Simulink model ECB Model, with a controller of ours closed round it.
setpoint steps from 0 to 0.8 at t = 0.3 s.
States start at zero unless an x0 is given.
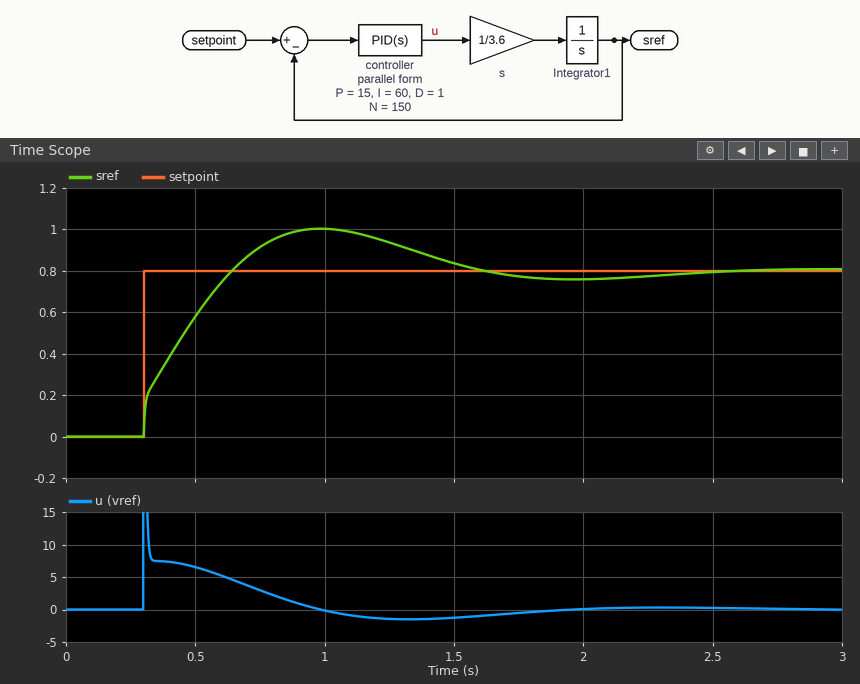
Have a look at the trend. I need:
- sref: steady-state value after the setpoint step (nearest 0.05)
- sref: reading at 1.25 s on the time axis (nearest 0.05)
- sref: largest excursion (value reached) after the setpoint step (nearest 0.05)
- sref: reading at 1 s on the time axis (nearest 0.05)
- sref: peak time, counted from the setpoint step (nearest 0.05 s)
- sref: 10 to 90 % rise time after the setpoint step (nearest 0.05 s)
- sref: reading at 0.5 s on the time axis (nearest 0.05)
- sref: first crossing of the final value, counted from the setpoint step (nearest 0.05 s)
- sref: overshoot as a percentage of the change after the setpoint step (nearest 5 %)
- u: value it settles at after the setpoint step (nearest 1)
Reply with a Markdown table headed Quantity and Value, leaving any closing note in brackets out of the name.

| Quantity | Value |
|---|---|
| sref: steady-state value after the setpoint step | 0.80 |
| sref: reading at 1.25 s on the time axis | 0.95 |
| sref: largest excursion (value reached) after the setpoint step | 1.00 |
| sref: reading at 1 s on the time axis | 1.00 |
| sref: peak time, counted from the setpoint step | 0.70 s |
| sref: 10 to 90 % rise time after the setpoint step | 0.30 s |
| sref: reading at 0.5 s on the time axis | 0.60 |
| sref: first crossing of the final value, counted from the setpoint step | 0.35 s |
| sref: overshoot as a percentage of the change after the setpoint step | 25 % |
| u: value it settles at after the setpoint step | 0 |
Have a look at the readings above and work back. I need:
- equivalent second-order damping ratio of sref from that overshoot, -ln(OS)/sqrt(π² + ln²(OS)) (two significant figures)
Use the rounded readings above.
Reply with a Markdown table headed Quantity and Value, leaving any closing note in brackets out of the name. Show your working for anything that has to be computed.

| Quantity | Value |
|---|---|
| equivalent second-order damping ratio of sref from that overshoot, -ln(OS)/sqrt(π² + ln²(OS)) | ln(0.25) = -1.386; 1.386 / sqrt(9.870 + 1.922) = 0.40 |
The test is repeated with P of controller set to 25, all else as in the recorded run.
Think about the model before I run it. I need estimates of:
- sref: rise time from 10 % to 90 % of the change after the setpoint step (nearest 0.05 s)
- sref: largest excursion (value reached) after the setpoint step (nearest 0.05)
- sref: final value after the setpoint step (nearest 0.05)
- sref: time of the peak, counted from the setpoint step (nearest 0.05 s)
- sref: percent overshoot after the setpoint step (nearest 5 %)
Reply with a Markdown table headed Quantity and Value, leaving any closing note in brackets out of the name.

| Quantity | Value |
|---|---|
| sref: rise time from 10 % to 90 % of the change after the setpoint step | 0.25 s |
| sref: largest excursion (value reached) after the setpoint step | 0.90 |
| sref: final value after the setpoint step | 0.80 |
| sref: time of the peak, counted from the setpoint step | 0.60 s |
| sref: percent overshoot after the setpoint step | 15 % |
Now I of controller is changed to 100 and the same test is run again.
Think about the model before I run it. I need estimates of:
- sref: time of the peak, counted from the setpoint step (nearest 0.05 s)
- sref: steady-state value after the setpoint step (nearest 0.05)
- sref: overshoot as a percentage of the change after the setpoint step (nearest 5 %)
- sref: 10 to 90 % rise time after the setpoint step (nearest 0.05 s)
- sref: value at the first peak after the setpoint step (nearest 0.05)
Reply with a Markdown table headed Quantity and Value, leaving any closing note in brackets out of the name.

| Quantity | Value |
|---|---|
| sref: time of the peak, counted from the setpoint step | 0.55 s |
| sref: steady-state value after the setpoint step | 0.80 |
| sref: overshoot as a percentage of the change after the setpoint step | 30 % |
| sref: 10 to 90 % rise time after the setpoint step | 0.25 s |
| sref: value at the first peak after the setpoint step | 1.05 |
